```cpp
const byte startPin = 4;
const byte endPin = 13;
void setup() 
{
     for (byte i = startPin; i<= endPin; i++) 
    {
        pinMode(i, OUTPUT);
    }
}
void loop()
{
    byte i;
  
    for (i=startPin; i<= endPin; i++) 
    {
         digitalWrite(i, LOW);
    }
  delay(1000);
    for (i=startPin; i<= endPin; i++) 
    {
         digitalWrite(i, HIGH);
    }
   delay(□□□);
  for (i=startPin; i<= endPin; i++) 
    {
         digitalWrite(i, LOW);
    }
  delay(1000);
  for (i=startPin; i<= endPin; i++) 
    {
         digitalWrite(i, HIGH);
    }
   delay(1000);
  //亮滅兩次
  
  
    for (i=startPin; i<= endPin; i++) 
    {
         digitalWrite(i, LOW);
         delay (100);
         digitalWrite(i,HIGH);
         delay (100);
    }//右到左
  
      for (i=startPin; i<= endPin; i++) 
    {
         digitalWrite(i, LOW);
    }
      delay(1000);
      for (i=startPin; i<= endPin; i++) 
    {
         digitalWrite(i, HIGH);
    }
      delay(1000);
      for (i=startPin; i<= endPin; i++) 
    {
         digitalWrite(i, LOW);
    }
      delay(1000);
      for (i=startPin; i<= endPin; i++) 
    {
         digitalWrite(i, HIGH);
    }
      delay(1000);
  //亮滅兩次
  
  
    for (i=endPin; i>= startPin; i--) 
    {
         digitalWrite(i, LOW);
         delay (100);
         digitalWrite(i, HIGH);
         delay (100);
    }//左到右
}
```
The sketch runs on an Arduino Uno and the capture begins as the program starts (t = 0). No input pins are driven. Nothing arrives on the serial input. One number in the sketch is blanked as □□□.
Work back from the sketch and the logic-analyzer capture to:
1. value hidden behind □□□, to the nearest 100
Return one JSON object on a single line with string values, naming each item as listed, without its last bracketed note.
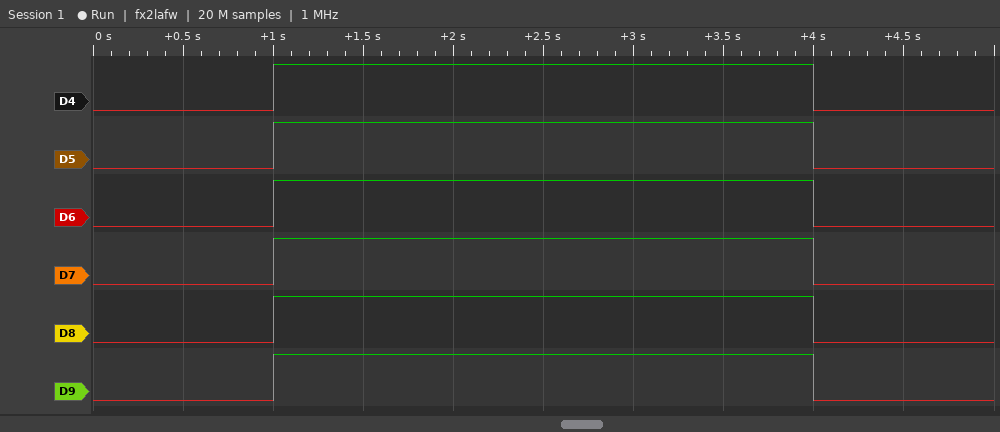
{"value hidden behind □□□, to the nearest 100": "3000"}
